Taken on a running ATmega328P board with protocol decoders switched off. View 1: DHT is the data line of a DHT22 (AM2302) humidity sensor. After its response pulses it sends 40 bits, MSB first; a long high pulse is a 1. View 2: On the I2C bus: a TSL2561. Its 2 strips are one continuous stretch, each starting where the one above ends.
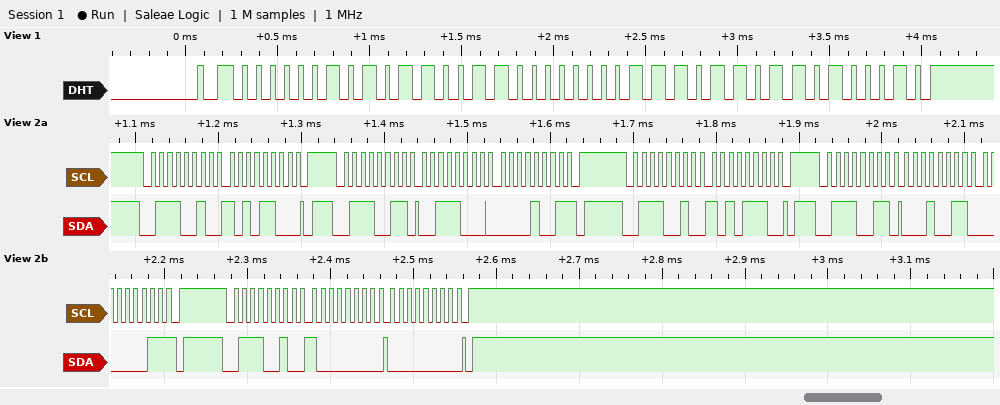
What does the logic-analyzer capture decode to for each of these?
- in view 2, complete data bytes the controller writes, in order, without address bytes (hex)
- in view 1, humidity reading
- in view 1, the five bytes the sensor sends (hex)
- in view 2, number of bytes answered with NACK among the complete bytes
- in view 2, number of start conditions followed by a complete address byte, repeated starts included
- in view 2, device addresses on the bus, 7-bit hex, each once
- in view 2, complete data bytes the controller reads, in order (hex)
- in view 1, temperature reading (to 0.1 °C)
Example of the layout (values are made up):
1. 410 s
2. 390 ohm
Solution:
1. AC AE 80 00
2. 69.1 %
3. 02 B3 00 ED A2
4. 2
5. 5
6. 0x39
7. 38 09 13 03
8. 23.7 °C
